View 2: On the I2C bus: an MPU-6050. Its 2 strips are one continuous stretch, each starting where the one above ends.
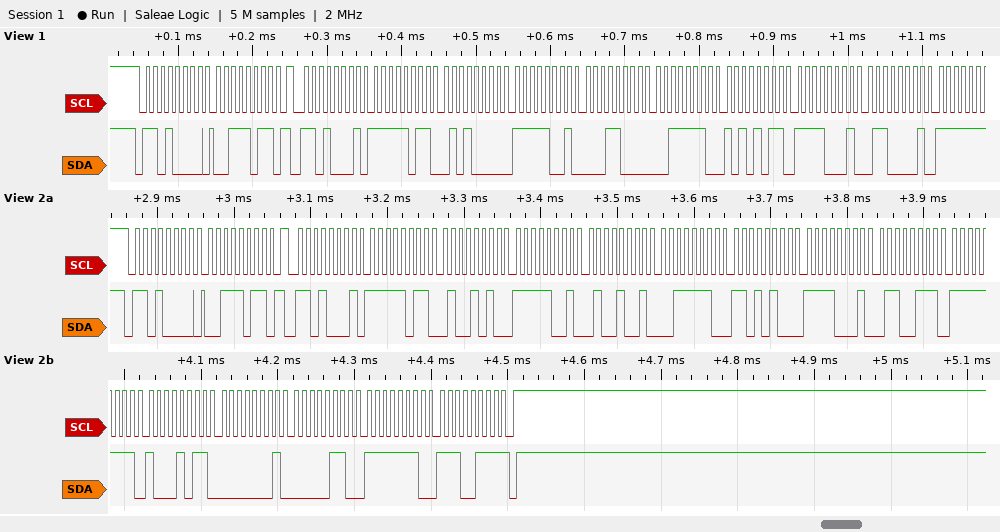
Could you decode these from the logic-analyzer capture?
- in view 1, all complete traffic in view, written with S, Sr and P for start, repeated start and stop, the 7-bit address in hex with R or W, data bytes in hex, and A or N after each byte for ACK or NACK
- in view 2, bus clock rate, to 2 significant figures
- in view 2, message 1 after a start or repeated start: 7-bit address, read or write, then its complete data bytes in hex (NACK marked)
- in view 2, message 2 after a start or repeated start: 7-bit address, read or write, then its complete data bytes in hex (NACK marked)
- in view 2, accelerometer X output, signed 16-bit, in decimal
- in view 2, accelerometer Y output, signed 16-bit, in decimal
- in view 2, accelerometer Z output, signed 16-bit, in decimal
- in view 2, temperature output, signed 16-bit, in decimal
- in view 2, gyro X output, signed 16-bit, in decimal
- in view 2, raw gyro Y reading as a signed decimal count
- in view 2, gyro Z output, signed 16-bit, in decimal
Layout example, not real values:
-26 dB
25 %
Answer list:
S 68W A 3B A Sr 68R A FB A 50 A F9 A 18 A 3E A AB A F1 A 61 A
100 kHz
0x68 write: 3B
0x68 read: FB 4A F9 49 3E D4 F1 67 FF 8B 01 06 FE E7 NACK
-1206
-1719
16084
-3737
-117
262
-281
